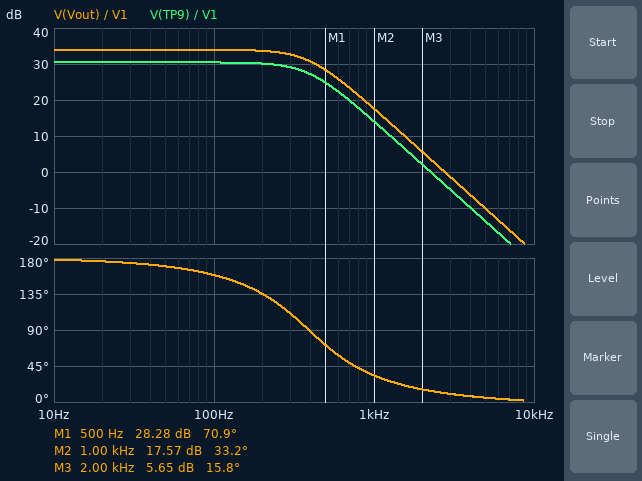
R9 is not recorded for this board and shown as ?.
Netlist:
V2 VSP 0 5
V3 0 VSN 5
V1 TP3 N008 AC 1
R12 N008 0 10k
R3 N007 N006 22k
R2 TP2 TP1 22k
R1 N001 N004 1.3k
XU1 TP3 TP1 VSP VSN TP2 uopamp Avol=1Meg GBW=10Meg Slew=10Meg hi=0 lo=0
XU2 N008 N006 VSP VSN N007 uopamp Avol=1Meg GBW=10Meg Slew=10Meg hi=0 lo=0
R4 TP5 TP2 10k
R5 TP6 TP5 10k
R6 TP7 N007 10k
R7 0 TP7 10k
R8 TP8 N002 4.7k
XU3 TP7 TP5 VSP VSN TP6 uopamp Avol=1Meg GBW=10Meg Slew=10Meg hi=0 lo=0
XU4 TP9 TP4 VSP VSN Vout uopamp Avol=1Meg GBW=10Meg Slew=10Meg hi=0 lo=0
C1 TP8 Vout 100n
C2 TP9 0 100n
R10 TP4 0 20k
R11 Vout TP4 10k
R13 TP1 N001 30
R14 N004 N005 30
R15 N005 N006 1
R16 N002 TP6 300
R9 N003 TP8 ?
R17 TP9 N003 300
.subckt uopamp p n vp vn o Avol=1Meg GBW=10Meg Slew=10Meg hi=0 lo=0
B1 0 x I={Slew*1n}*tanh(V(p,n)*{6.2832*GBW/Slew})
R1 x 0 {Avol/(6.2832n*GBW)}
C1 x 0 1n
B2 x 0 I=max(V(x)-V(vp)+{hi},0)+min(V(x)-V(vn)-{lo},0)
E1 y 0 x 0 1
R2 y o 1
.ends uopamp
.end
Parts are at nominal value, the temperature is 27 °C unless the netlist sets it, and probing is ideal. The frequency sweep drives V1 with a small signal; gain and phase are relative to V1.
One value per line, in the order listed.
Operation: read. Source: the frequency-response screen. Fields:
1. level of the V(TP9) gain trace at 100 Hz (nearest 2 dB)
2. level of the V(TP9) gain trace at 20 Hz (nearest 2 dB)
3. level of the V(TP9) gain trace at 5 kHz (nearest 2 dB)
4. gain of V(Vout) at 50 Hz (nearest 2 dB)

30 dB
30 dB
-14 dB
34 dB
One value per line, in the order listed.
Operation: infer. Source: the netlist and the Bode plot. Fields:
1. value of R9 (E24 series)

3 kΩ
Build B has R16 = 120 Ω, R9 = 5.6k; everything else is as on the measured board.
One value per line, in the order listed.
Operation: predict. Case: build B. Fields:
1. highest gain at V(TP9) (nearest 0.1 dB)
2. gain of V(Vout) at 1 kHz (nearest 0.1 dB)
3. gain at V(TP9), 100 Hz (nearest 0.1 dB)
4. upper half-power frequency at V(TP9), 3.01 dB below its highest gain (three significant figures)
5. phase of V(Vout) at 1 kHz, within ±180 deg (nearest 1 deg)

30.5 dB
12.8 dB
30.2 dB
268 Hz
27 deg
